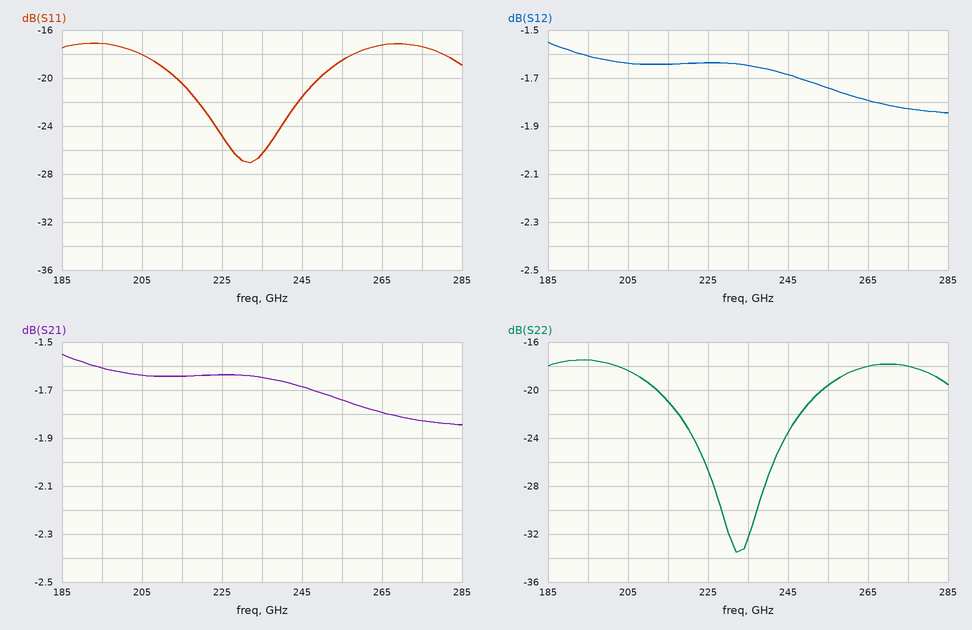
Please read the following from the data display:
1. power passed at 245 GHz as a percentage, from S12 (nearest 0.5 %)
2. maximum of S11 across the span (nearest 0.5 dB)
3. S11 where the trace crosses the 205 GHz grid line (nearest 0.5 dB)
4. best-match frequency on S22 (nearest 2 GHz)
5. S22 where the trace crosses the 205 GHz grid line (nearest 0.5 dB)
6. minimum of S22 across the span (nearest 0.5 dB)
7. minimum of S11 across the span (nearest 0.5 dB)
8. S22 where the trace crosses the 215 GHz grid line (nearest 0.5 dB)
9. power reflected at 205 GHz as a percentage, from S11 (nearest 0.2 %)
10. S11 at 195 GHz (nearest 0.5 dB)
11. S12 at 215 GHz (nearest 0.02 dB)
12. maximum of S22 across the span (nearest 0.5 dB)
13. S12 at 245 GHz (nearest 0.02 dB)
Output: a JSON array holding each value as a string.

["68.0 %", "-17.0 dB", "-18.0 dB", "232 GHz", "-18.5 dB", "-33.5 dB", "-27.0 dB", "-21.0 dB", "1.6 %", "-17.0 dB", "-1.64 dB", "-17.5 dB", "-1.68 dB"]
